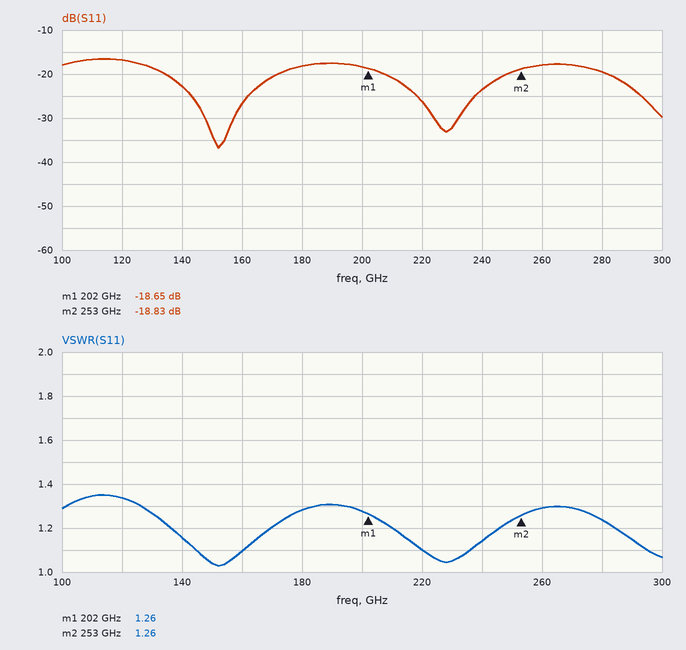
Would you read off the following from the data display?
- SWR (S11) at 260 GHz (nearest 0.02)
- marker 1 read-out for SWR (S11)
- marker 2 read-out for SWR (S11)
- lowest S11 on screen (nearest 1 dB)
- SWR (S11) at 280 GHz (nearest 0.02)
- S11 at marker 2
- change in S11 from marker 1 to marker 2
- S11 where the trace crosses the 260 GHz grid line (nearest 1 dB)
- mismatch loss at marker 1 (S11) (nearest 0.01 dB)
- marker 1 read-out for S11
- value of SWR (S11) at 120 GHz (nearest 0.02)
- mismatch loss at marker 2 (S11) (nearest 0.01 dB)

1.30
1.26
1.26
-37 dB
1.24
-18.83 dB
-0.18 dB
-18 dB
0.06 dB
-18.65 dB
1.34
0.06 dB
